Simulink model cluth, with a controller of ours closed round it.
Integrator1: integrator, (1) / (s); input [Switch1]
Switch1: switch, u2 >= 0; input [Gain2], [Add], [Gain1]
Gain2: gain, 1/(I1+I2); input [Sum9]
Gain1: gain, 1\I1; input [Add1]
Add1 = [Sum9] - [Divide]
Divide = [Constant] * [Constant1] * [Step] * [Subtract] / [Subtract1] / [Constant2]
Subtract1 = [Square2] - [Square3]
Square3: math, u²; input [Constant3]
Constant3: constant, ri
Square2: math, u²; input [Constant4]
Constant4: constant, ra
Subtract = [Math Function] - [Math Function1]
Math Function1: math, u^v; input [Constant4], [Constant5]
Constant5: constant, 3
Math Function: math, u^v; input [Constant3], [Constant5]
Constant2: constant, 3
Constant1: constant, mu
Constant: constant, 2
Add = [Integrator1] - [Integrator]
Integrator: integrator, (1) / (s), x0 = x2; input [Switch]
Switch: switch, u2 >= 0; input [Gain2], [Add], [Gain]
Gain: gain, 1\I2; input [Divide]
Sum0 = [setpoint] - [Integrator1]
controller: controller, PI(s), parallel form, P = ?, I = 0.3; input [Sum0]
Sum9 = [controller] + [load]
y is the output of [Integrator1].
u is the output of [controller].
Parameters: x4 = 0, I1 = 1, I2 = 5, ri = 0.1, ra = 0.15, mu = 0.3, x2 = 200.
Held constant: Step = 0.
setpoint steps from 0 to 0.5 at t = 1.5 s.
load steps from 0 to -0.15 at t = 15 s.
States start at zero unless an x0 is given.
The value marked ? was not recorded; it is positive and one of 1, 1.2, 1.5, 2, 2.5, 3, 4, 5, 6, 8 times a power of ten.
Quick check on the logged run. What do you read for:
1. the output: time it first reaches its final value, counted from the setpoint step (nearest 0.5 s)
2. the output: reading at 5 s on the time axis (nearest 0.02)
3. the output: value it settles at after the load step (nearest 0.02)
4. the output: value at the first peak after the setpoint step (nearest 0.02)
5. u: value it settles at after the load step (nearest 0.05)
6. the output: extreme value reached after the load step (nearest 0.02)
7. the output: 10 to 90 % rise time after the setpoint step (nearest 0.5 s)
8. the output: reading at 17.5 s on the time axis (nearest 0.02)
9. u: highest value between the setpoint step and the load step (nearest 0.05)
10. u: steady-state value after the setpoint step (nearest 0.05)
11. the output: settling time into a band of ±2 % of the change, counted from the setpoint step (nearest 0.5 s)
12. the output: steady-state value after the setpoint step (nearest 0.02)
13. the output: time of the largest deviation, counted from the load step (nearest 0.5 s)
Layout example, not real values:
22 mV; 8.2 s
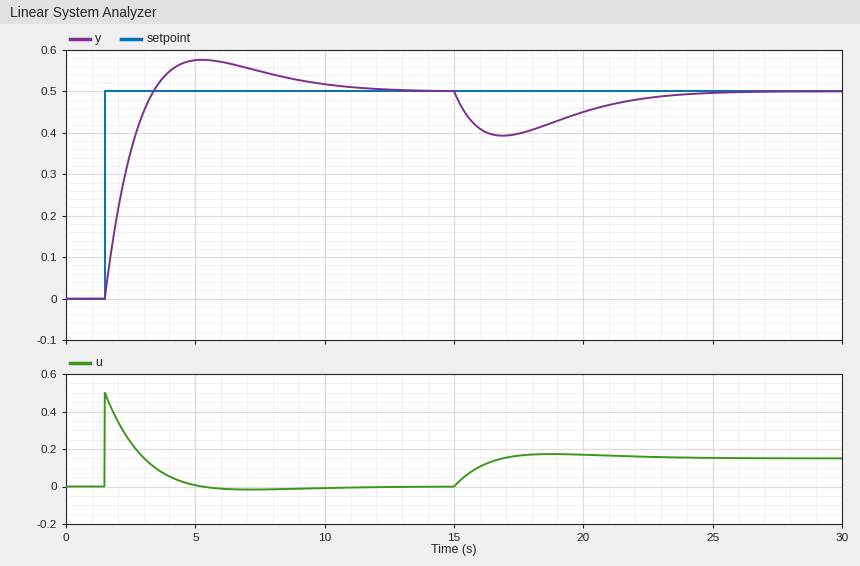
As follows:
2.0 s; 0.58; 0.50; 0.58; 0.15; 0.40; 1.5 s; 0.40; 0.50; 0.00; 9.5 s; 0.50; 2.0 s
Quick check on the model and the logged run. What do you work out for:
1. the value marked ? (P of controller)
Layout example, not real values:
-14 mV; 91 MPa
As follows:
1
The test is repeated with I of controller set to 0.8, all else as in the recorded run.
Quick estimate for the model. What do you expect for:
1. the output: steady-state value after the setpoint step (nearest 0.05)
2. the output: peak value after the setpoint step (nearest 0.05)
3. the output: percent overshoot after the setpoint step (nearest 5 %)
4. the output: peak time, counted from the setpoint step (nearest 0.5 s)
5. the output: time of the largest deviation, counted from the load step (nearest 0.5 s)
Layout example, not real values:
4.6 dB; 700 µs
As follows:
0.50; 0.65; 25 %; 2.5 s; 1.5 s
